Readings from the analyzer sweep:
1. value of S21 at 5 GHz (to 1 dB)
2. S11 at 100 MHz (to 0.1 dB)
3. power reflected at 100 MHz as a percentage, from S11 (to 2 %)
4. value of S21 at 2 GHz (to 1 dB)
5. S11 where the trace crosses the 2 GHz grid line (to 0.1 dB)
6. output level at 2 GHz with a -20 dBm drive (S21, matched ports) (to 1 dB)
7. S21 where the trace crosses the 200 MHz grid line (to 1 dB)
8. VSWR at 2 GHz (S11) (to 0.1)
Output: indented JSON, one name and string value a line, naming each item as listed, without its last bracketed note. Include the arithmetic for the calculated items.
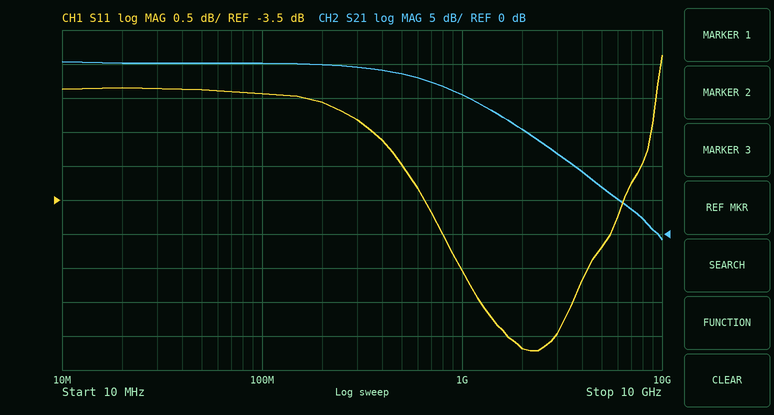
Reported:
{
  "value of S21 at 5 GHz": "7 dB",
  "S11 at 100 MHz": "-1.9 dB",
  "power reflected at 100 MHz as a percentage, from S11": "10^(-1.9/10) ≈ 64.6 %, so 64 % to the nearest 2 %",
  "value of S21 at 2 GHz": "15 dB",
  "S11 where the trace crosses the 2 GHz grid line": "-5.7 dB",
  "output level at 2 GHz with a -20 dBm drive (S21, matched ports)": "-20 dBm + (15 dB) = -5 dBm",
  "S21 where the trace crosses the 200 MHz grid line": "25 dB",
  "VSWR at 2 GHz (S11)": "|Γ| = 10^(-5.7/20) = 0.5188; VSWR = (1 + 0.5188)/(1 − 0.5188) ≈ 3.2"
}
